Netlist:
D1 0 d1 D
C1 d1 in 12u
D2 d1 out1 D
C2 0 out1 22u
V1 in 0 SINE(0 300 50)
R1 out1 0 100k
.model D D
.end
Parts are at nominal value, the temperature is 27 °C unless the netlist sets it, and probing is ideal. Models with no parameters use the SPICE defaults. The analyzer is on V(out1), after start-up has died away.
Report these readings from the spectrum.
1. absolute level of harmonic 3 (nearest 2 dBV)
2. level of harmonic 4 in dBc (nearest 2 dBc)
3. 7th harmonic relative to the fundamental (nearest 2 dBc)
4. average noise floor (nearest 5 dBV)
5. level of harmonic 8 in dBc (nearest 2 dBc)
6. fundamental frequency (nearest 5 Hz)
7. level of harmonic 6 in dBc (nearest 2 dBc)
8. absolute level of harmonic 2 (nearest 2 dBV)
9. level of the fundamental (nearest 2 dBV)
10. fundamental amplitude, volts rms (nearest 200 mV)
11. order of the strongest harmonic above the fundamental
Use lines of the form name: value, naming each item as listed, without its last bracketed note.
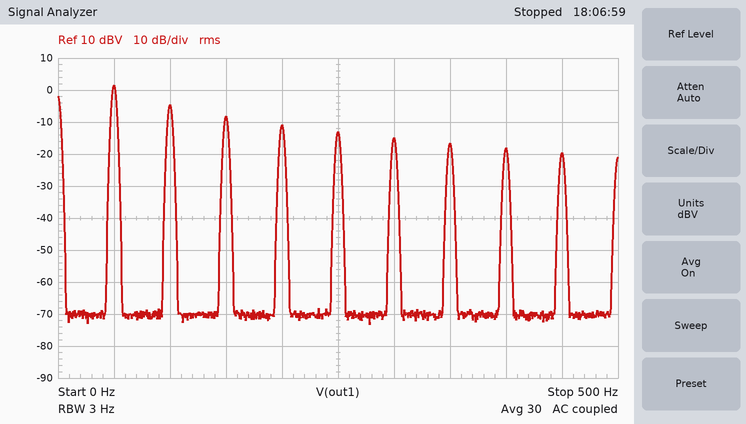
absolute level of harmonic 3: -8 dBV
level of harmonic 4 in dBc: -12 dBc
7th harmonic relative to the fundamental: -18 dBc
average noise floor: -70 dBV
level of harmonic 8 in dBc: -20 dBc
fundamental frequency: 50 Hz
level of harmonic 6 in dBc: -16 dBc
absolute level of harmonic 2: -4 dBV
level of the fundamental: 2 dBV
fundamental amplitude, volts rms: 1.2 V
order of the strongest harmonic above the fundamental: 2
